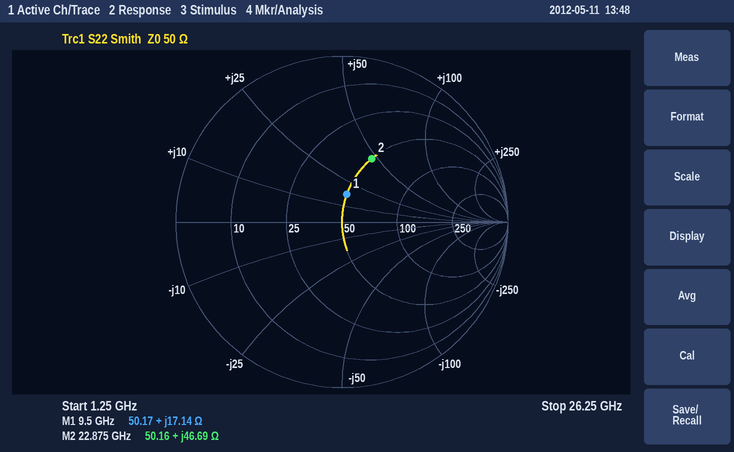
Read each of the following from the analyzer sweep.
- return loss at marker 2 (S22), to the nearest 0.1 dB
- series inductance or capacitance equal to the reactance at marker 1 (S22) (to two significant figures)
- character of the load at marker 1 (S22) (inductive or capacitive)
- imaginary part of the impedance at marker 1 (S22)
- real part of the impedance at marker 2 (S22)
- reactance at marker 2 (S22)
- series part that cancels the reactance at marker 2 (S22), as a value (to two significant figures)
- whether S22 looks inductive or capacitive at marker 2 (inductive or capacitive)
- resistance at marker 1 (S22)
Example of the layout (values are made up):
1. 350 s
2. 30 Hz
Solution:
1. 7.5 dB
2. 290 pH
3. inductive
4. +17.14 Ω
5. 50.16 Ω
6. +46.69 Ω
7. 150 fF
8. inductive
9. 50.17 Ω
